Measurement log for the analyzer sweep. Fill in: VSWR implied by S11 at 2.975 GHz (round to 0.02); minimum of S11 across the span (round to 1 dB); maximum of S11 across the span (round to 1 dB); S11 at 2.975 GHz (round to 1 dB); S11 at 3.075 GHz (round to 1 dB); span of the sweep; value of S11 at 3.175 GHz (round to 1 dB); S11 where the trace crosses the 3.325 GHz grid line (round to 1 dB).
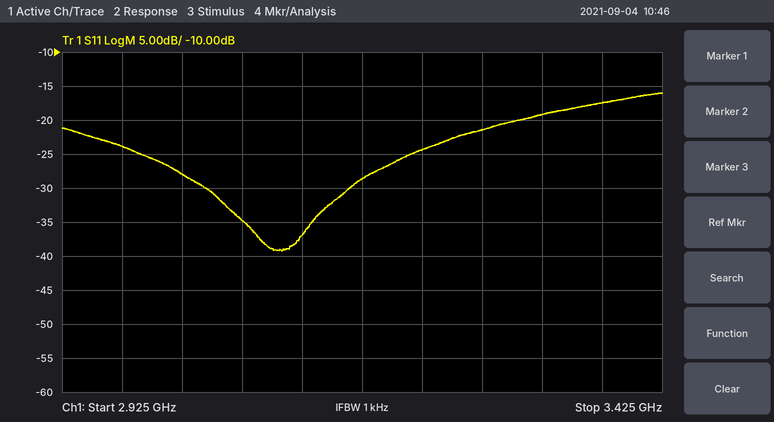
1.14
-39 dB
-16 dB
-24 dB
-35 dB
500 MHz
-29 dB
-19 dB
